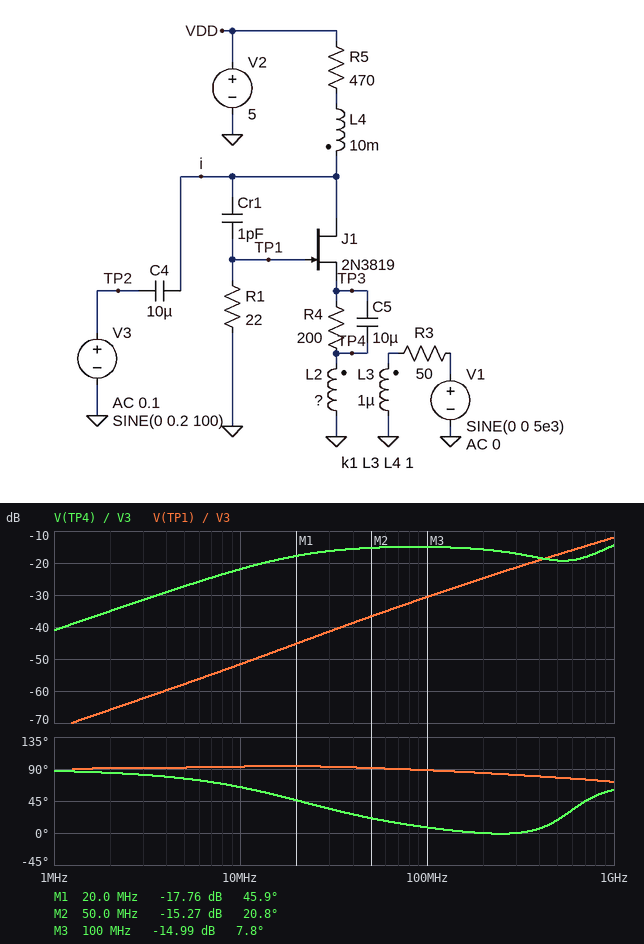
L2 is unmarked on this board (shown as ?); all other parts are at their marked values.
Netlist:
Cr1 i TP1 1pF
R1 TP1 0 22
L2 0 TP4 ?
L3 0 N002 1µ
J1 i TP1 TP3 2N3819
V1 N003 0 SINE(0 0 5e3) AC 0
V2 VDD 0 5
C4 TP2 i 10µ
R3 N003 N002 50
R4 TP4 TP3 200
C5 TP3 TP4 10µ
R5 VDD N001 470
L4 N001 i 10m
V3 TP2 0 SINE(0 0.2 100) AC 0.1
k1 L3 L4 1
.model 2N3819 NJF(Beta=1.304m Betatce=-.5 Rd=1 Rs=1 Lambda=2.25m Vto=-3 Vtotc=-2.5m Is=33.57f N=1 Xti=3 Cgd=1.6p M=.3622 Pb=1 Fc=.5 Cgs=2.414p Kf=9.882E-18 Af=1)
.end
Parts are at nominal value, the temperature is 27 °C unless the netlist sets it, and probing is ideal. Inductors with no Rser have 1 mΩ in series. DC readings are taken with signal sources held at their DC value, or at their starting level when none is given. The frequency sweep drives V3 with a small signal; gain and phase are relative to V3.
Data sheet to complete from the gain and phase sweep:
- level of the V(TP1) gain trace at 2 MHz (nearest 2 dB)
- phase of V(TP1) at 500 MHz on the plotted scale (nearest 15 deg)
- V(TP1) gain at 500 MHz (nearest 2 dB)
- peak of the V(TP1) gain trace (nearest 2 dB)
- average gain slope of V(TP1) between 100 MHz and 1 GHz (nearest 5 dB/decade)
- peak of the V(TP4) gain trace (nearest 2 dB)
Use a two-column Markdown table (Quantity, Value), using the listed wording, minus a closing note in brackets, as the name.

| Quantity | Value |
|---|---|
| level of the V(TP1) gain trace at 2 MHz | -66 dB |
| phase of V(TP1) at 500 MHz on the plotted scale | 75 deg |
| V(TP1) gain at 500 MHz | -18 dB |
| peak of the V(TP1) gain trace | -12 dB |
| average gain slope of V(TP1) between 100 MHz and 1 GHz | 20 dB/decade |
| peak of the V(TP4) gain trace | -14 dB |
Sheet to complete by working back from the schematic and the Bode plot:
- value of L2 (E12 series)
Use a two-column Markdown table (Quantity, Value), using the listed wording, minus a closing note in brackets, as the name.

| Quantity | Value |
|---|---|
| value of L2 | 1.5 µH |
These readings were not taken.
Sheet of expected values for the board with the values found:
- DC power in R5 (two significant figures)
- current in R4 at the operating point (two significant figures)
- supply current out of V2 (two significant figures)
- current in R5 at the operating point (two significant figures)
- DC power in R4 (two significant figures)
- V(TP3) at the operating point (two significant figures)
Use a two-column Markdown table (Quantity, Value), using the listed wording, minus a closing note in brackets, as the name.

| Quantity | Value |
|---|---|
| DC power in R5 | 12 mW |
| current in R4 at the operating point | 5.0 mA |
| supply current out of V2 | 5.0 mA |
| current in R5 at the operating point | 5.0 mA |
| DC power in R4 | 5.0 mW |
| V(TP3) at the operating point | 1.0 V |
